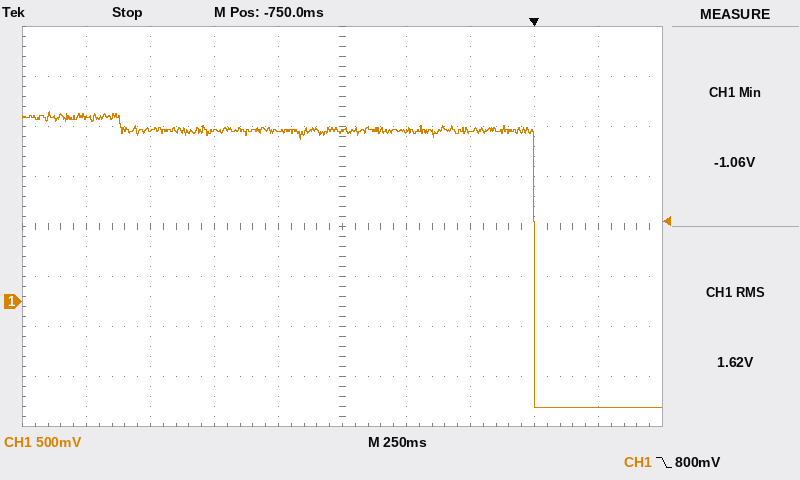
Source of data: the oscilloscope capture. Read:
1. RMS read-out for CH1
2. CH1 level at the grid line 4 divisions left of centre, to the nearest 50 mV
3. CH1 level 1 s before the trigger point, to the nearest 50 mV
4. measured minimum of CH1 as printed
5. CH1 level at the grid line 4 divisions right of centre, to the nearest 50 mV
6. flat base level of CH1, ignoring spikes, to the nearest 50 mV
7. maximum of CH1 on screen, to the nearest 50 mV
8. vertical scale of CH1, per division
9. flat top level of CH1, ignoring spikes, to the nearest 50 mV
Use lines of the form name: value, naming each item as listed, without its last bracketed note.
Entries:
RMS read-out for CH1: 1.62 V
CH1 level at the grid line 4 divisions left of centre, to the nearest 50 mV: 1.85 V
CH1 level 1 s before the trigger point, to the nearest 50 mV: 1.70 V
measured minimum of CH1 as printed: -1.06 V
CH1 level at the grid line 4 divisions right of centre, to the nearest 50 mV: -1.05 V
flat base level of CH1, ignoring spikes, to the nearest 50 mV: -1.05 V
maximum of CH1 on screen, to the nearest 50 mV: 1.90 V
vertical scale of CH1, per division: 500 mV
flat top level of CH1, ignoring spikes, to the nearest 50 mV: 1.70 V
